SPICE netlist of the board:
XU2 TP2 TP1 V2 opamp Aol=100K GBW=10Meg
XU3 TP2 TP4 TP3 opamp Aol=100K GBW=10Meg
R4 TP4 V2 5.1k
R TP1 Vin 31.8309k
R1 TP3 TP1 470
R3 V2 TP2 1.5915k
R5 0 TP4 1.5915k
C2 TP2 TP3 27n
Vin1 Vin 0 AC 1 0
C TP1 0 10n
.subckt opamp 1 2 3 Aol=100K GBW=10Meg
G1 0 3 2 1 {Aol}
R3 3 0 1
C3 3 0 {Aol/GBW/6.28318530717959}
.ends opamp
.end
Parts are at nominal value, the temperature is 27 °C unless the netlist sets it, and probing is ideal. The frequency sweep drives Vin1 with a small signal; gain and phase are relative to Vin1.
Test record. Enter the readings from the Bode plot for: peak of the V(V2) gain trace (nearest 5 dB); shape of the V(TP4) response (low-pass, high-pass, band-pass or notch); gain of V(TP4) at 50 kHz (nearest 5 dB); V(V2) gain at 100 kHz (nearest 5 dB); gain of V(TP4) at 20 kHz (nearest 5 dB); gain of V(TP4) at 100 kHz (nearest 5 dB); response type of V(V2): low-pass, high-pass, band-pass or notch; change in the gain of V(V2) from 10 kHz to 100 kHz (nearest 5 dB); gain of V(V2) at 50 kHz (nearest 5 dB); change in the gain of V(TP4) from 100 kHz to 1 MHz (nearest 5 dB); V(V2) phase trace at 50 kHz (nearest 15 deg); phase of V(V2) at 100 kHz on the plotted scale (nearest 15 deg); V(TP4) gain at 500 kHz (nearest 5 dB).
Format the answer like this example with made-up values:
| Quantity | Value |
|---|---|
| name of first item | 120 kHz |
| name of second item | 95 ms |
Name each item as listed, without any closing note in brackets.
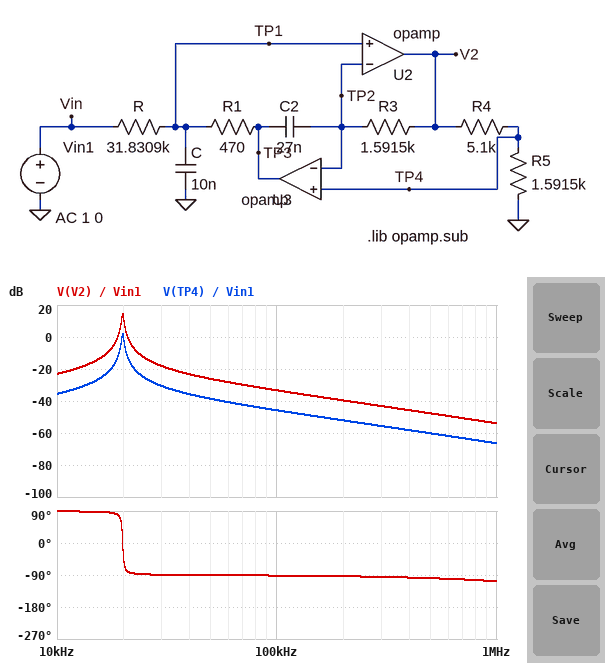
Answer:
| Quantity | Value |
|---|---|
| peak of the V(V2) gain trace | 15 dB |
| shape of the V(TP4) response | band-pass |
| gain of V(TP4) at 50 kHz | -40 dB |
| V(V2) gain at 100 kHz | -35 dB |
| gain of V(TP4) at 20 kHz | 0 dB |
| gain of V(TP4) at 100 kHz | -45 dB |
| response type of V(V2): low-pass, high-pass, band-pass or notch | band-pass |
| change in the gain of V(V2) from 10 kHz to 100 kHz | -10 dB |
| gain of V(V2) at 50 kHz | -25 dB |
| change in the gain of V(TP4) from 100 kHz to 1 MHz | -20 dB |
| V(V2) phase trace at 50 kHz | -90 deg |
| phase of V(V2) at 100 kHz on the plotted scale | -90 deg |
| V(TP4) gain at 500 kHz | -60 dB |
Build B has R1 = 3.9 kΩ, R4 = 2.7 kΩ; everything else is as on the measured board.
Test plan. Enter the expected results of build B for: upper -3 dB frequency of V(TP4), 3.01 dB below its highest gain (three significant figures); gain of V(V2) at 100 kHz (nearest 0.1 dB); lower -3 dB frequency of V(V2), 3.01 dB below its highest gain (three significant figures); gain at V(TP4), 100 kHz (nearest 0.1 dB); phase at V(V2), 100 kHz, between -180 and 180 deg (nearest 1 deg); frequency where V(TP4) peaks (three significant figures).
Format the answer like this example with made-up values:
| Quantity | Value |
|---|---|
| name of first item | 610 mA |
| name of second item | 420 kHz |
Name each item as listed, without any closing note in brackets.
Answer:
| Quantity | Value |
|---|---|
| upper -3 dB frequency of V(TP4), 3.01 dB below its highest gain | 5.31 kHz |
| gain of V(V2) at 100 kHz | -37.4 dB |
| lower -3 dB frequency of V(V2), 3.01 dB below its highest gain | 4.82 kHz |
| gain at V(TP4), 100 kHz | -46.0 dB |
| phase at V(V2), 100 kHz, between -180 and 180 deg | -91 deg |
| frequency where V(TP4) peaks | 5.06 kHz |
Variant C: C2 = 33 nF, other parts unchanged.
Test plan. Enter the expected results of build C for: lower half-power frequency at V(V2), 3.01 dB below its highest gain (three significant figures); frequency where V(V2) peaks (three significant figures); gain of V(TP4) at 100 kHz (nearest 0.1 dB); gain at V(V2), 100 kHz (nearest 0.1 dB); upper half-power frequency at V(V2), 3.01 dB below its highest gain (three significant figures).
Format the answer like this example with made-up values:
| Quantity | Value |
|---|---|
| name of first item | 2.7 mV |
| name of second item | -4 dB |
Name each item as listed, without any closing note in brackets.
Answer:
| Quantity | Value |
|---|---|
| lower half-power frequency at V(V2), 3.01 dB below its highest gain | 17.8 kHz |
| frequency where V(V2) peaks | 18.0 kHz |
| gain of V(TP4) at 100 kHz | -45.9 dB |
| gain at V(V2), 100 kHz | -33.4 dB |
| upper half-power frequency at V(V2), 3.01 dB below its highest gain | 18.2 kHz |
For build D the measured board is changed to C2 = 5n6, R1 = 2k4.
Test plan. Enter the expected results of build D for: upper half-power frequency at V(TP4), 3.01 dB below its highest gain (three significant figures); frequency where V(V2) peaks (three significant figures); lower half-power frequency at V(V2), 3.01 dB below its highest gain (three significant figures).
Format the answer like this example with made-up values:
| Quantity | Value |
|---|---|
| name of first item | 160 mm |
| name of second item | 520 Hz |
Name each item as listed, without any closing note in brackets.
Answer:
| Quantity | Value |
|---|---|
| upper half-power frequency at V(TP4), 3.01 dB below its highest gain | 19.6 kHz |
| frequency where V(V2) peaks | 19.4 kHz |
| lower half-power frequency at V(V2), 3.01 dB below its highest gain | 19.2 kHz |
